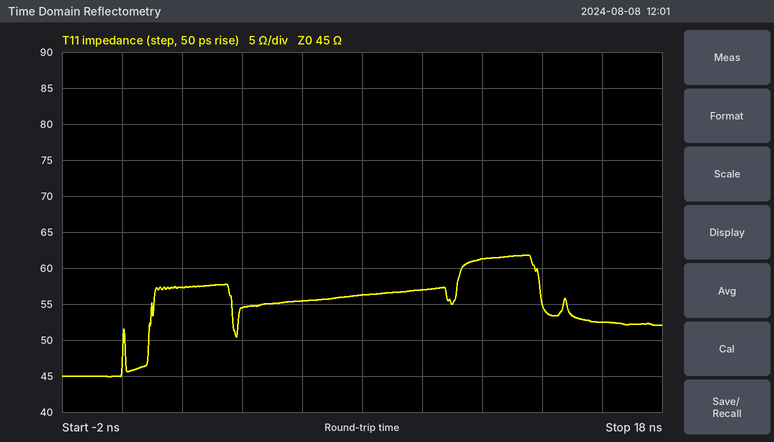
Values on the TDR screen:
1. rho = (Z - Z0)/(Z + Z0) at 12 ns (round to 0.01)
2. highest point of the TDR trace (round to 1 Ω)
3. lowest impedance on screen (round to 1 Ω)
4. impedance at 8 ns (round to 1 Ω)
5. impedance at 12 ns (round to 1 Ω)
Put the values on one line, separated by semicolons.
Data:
+0.15; 62 Ω; 45 Ω; 56 Ω; 61 Ω
